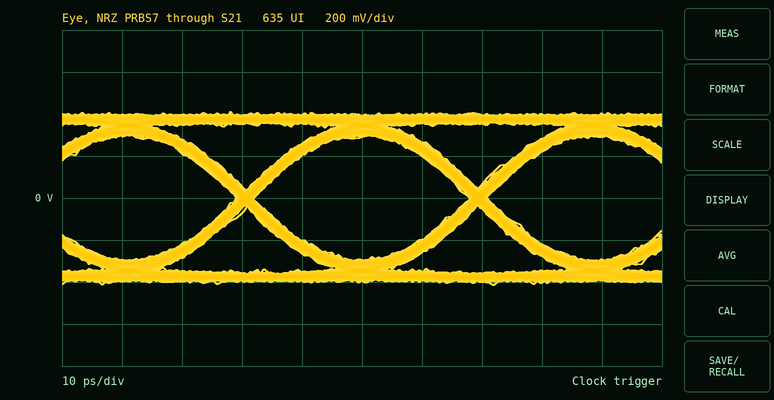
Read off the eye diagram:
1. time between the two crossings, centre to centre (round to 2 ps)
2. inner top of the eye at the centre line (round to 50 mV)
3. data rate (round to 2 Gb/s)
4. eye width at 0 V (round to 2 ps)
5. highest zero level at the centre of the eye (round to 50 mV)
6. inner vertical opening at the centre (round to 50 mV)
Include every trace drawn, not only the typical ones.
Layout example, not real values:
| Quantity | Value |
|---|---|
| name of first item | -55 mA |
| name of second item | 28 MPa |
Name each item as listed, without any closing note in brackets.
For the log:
| Quantity | Value |
|---|---|
| time between the two crossings, centre to centre | 38 ps |
| inner top of the eye at the centre line | 300 mV |
| data rate | 26 Gb/s |
| eye width at 0 V | 36 ps |
| highest zero level at the centre of the eye | -300 mV |
| inner vertical opening at the centre | 600 mV |
